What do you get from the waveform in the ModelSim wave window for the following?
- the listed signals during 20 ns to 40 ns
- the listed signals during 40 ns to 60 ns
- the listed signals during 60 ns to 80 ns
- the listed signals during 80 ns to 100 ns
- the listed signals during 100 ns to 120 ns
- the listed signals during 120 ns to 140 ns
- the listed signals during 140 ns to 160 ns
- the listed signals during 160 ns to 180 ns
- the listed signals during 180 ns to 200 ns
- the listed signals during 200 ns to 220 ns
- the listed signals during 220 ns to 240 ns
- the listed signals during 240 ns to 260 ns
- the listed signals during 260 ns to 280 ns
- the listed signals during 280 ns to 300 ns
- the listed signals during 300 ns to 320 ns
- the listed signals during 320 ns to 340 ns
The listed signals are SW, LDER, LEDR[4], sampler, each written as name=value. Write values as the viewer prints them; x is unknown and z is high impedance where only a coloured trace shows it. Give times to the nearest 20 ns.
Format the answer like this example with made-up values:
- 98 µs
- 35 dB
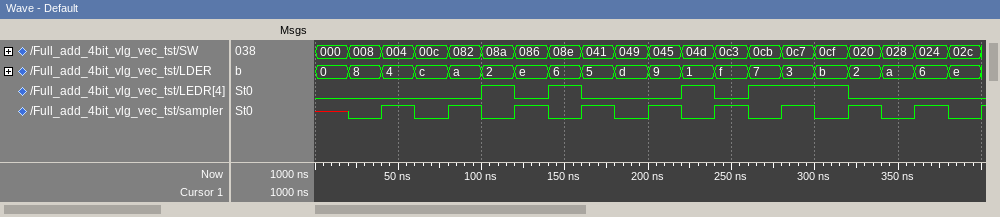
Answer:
- SW=008, LDER=8, LEDR[4]=0, sampler=0
- SW=004, LDER=4, LEDR[4]=0, sampler=1
- SW=00c, LDER=c, LEDR[4]=0, sampler=0
- SW=082, LDER=a, LEDR[4]=0, sampler=1
- SW=08a, LDER=2, LEDR[4]=1, sampler=0
- SW=086, LDER=e, LEDR[4]=0, sampler=1
- SW=08e, LDER=6, LEDR[4]=1, sampler=0
- SW=041, LDER=5, LEDR[4]=0, sampler=1
- SW=049, LDER=d, LEDR[4]=0, sampler=0
- SW=045, LDER=9, LEDR[4]=0, sampler=1
- SW=04d, LDER=1, LEDR[4]=1, sampler=0
- SW=0c3, LDER=f, LEDR[4]=0, sampler=1
- SW=0cb, LDER=7, LEDR[4]=1, sampler=0
- SW=0c7, LDER=3, LEDR[4]=1, sampler=1
- SW=0cf, LDER=b, LEDR[4]=1, sampler=0
- SW=020, LDER=2, LEDR[4]=0, sampler=1
